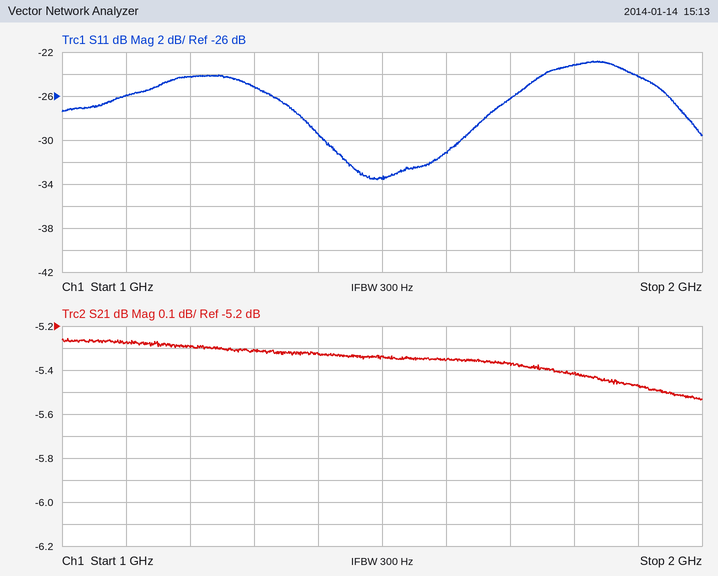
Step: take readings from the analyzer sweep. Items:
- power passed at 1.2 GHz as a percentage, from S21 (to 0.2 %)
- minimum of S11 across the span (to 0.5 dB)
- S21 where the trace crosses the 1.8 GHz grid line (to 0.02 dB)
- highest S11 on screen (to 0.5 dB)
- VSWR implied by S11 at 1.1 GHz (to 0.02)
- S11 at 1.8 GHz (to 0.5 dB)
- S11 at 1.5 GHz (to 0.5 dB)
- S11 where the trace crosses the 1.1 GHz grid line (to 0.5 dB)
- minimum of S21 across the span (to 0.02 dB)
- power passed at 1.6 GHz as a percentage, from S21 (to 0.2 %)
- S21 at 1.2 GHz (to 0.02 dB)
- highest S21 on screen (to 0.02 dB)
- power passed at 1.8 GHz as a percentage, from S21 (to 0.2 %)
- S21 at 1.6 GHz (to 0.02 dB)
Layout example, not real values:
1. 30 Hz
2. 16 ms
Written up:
1. 29.6 %
2. -33.5 dB
3. -5.42 dB
4. -23.0 dB
5. 1.10
6. -23.0 dB
7. -33.5 dB
8. -26.0 dB
9. -5.54 dB
10. 29.2 %
11. -5.30 dB
12. -5.26 dB
13. 28.8 %
14. -5.36 dB
